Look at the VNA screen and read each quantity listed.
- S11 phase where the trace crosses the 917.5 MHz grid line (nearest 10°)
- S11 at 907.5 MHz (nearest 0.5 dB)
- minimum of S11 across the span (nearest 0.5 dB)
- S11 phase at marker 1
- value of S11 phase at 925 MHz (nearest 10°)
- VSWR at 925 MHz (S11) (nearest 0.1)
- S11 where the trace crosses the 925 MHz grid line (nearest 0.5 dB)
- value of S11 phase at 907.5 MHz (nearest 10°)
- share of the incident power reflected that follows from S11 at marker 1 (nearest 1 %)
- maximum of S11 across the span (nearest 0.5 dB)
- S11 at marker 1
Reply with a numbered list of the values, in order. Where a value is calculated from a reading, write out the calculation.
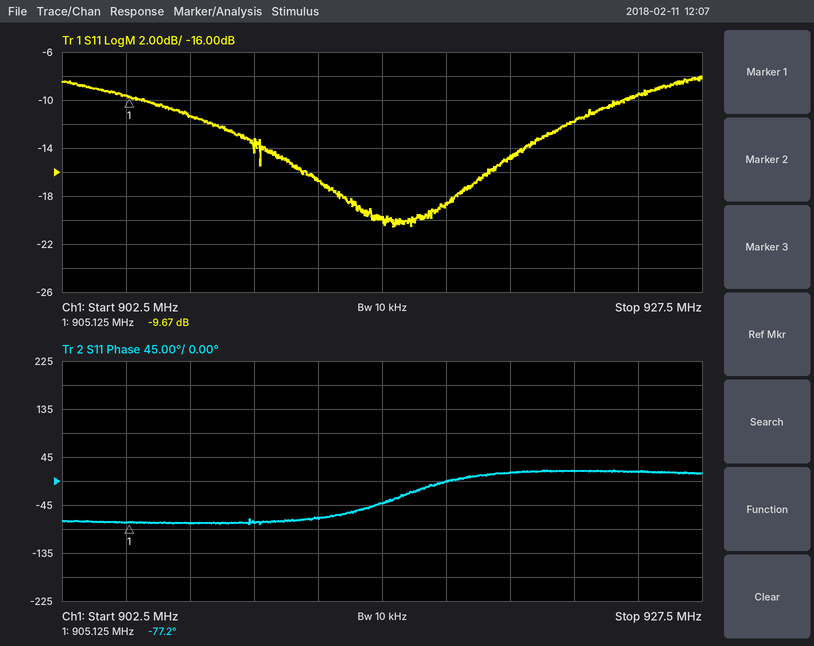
1. 0°
2. -11.5 dB
3. -20.5 dB
4. -77.2°
5. 20°
6. |Γ| = 10^(-9.5/20) = 0.3350; VSWR = (1 + 0.3350)/(1 − 0.3350) ≈ 2.0
7. -9.5 dB
8. -80°
9. 10^(-9.67/10) ≈ 11 %
10. -8.0 dB
11. -9.67 dB
